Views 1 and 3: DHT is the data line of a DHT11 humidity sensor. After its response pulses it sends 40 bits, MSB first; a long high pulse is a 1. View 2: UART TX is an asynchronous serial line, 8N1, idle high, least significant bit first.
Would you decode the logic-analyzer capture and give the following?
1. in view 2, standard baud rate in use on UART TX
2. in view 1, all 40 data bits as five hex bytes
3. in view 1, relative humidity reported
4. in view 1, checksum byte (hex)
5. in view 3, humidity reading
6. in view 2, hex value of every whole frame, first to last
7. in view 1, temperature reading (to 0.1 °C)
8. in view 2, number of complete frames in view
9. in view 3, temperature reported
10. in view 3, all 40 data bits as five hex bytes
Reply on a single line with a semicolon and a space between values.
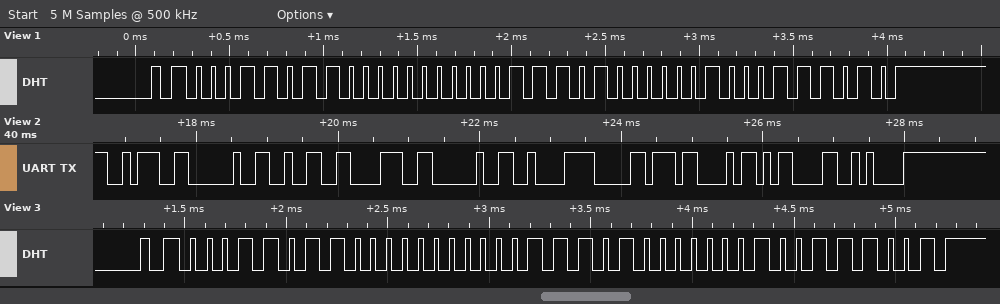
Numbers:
9600 baud; 1B 00 1D 02 3A; 27 %; 0x3A; 27 %; 3A 20 32 38 20 C2 B0 43 0D 0A; 29.2 °C; 10; 29.1 °C; 1B 00 1D 01 39
